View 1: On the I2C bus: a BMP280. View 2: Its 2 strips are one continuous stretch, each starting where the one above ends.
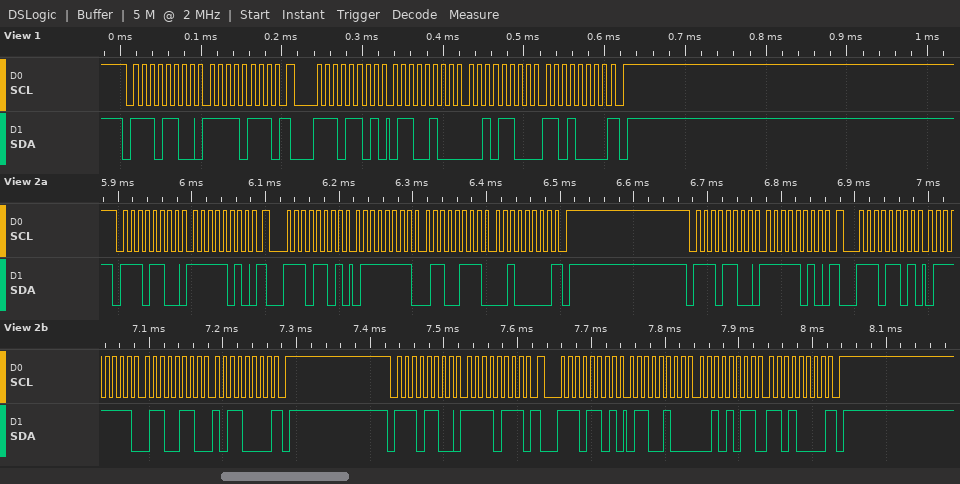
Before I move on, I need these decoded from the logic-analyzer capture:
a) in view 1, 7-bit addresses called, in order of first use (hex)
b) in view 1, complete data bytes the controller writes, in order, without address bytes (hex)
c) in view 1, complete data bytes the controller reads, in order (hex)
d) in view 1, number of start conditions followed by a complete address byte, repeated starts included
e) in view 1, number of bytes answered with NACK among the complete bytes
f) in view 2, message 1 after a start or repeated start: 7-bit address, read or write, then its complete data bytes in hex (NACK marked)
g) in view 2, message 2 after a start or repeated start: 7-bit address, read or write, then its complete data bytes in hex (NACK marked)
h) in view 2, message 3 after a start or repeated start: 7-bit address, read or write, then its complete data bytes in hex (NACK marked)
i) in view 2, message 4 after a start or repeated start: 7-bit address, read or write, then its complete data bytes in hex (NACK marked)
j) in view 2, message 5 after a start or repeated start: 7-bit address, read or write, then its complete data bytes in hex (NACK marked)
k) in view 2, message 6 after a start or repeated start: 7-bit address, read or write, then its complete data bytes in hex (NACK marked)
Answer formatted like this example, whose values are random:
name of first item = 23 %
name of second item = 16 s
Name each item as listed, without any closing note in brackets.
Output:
in view 1, 7-bit addresses called, in order of first use = 0x76
in view 1, complete data bytes the controller writes, in order, without address bytes = F7
in view 1, complete data bytes the controller reads, in order = 64 2C D0
in view 1, number of start conditions followed by a complete address byte, repeated starts included = 2
in view 1, number of bytes answered with NACK among the complete bytes = 1
in view 2, message 1 after a start or repeated start: 7-bit address, read or write, then its complete data bytes in hex = 0x76 write: FA
in view 2, message 2 after a start or repeated start: 7-bit address, read or write, then its complete data bytes in hex = 0x76 read: 7F 67 20 NACK
in view 2, message 3 after a start or repeated start: 7-bit address, read or write, then its complete data bytes in hex = 0x76 write: FA
in view 2, message 4 after a start or repeated start: 7-bit address, read or write, then its complete data bytes in hex = 0x76 read: 7F 66 B0 NACK
in view 2, message 5 after a start or repeated start: 7-bit address, read or write, then its complete data bytes in hex = 0x76 write: F7
in view 2, message 6 after a start or repeated start: 7-bit address, read or write, then its complete data bytes in hex = 0x76 read: 64 2B D0 NACK
